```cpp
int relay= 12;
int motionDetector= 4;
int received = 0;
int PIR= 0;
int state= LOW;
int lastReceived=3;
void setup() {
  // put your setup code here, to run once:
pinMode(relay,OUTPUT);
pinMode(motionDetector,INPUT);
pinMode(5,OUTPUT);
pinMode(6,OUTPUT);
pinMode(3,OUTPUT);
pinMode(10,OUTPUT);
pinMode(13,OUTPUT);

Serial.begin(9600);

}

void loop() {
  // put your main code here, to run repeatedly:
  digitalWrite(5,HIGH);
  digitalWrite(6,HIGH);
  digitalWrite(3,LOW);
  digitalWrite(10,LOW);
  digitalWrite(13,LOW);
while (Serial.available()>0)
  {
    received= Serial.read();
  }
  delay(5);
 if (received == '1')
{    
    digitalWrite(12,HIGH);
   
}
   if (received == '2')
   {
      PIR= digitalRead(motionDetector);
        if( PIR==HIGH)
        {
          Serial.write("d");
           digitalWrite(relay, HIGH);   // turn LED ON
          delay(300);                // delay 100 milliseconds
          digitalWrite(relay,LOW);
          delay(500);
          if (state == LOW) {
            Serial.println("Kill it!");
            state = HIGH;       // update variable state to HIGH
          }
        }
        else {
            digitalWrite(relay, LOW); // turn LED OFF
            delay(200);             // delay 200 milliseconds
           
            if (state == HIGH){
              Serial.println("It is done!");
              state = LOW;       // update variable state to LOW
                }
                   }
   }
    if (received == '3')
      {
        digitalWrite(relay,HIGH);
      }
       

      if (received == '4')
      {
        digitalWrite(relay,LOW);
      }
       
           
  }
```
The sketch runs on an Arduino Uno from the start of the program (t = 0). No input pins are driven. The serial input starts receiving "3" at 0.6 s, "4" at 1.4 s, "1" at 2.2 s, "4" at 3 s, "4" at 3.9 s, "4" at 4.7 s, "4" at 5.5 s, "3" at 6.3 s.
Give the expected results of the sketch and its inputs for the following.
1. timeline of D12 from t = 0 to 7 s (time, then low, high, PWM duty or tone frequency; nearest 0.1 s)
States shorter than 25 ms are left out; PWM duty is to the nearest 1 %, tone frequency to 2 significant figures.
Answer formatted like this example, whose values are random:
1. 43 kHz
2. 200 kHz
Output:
1. 0 s low; 0.6 s high; 1.4 s low; 2.2 s high; 3 s low; 6.3 s high
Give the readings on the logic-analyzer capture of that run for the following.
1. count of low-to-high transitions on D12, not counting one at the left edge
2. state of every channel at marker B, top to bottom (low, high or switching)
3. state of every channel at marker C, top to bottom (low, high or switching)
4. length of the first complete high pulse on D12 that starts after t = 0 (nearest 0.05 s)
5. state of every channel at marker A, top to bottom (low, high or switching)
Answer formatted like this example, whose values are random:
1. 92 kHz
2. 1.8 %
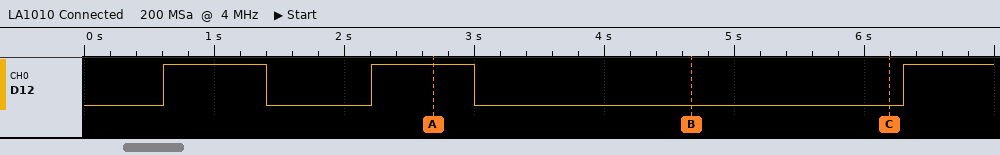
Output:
1. 3
2. D12 low
3. D12 low
4. 0.80 s
5. D12 high
